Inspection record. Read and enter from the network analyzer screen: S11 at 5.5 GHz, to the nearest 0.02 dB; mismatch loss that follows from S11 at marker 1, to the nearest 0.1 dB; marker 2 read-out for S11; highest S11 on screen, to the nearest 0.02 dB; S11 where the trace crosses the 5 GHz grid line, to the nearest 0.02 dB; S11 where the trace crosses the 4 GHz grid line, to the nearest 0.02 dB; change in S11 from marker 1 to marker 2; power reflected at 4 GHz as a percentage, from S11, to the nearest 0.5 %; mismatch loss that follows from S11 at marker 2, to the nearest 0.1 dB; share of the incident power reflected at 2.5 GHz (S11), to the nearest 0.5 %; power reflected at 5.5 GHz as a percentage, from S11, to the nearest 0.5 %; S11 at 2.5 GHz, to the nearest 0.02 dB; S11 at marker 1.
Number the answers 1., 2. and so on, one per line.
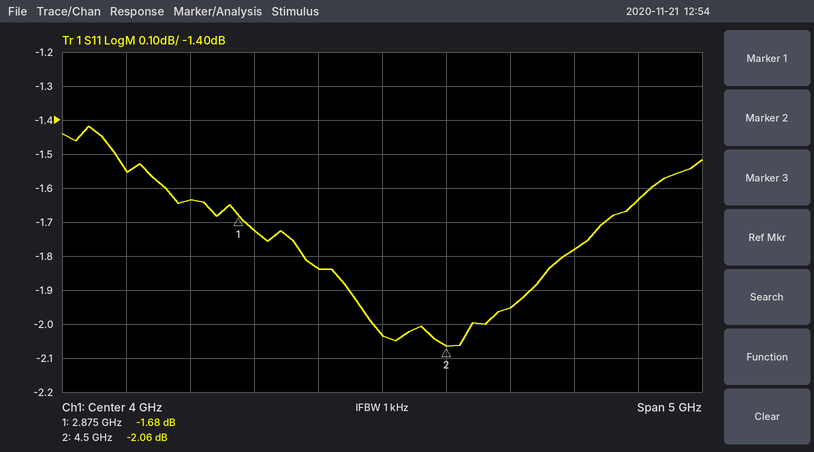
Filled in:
1. -1.78 dB
2. 4.9 dB
3. -2.06 dB
4. -1.42 dB
5. -1.96 dB
6. -2.04 dB
7. -0.38 dB
8. 62.5 %
9. 4.2 dB
10. 68.5 %
11. 66.5 %
12. -1.64 dB
13. -1.68 dB
